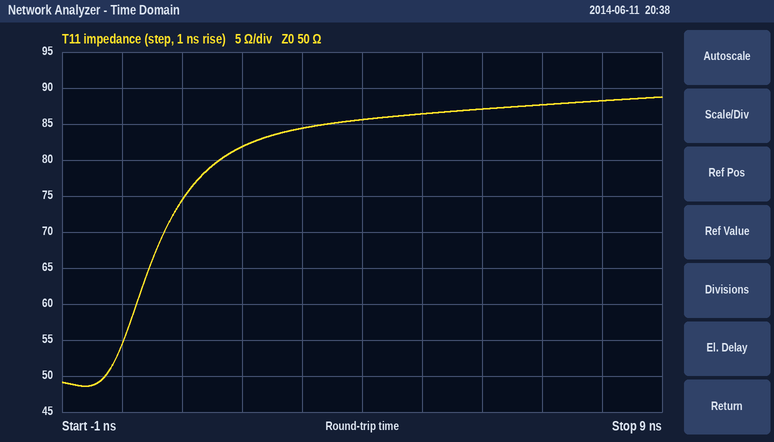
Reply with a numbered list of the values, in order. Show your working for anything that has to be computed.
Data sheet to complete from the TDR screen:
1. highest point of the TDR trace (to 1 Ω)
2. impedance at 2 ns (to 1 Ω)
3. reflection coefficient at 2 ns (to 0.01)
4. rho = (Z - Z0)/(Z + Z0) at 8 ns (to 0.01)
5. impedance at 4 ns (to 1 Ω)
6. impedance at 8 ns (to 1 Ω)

1. 89 Ω
2. 82 Ω
3. (82 − 50)/(82 + 50) ≈ +0.24
4. (88 − 50)/(88 + 50) ≈ +0.28
5. 86 Ω
6. 88 Ω
